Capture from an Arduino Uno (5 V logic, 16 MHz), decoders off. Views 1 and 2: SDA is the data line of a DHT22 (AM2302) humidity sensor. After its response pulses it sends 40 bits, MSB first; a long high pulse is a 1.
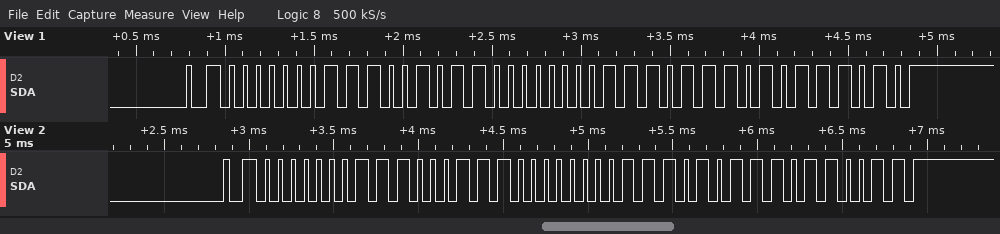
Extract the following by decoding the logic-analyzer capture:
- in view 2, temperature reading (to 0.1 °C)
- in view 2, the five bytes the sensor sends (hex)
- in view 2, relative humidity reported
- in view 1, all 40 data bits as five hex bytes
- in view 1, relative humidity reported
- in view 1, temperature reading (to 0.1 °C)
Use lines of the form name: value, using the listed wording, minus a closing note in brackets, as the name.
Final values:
in view 2, temperature reading: 23.5 °C
in view 2, the five bytes the sensor sends: 01 C7 00 EB B3
in view 2, relative humidity reported: 45.5 %
in view 1, all 40 data bits as five hex bytes: 01 CB 00 EE BA
in view 1, relative humidity reported: 45.9 %
in view 1, temperature reading: 23.8 °C
